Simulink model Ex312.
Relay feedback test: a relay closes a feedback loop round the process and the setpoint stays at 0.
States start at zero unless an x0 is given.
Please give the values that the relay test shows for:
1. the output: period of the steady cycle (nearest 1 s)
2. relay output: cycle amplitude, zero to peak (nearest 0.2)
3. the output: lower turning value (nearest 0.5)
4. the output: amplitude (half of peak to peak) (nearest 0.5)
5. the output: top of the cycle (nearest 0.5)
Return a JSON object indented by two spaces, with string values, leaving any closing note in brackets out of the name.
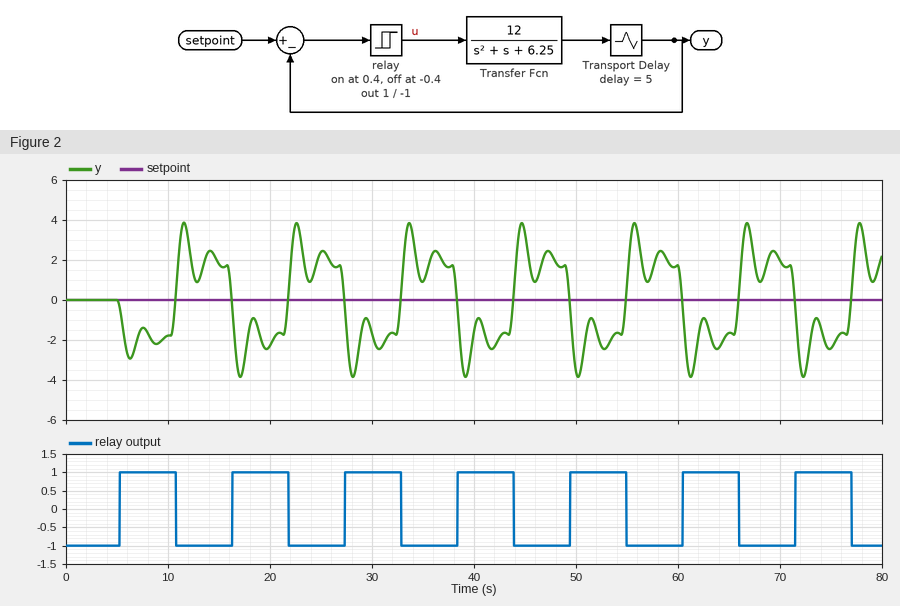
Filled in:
{
  "the output: period of the steady cycle": "11 s",
  "relay output: cycle amplitude, zero to peak": "1.0",
  "the output: lower turning value": "-4.0",
  "the output: amplitude (half of peak to peak)": "4.0",
  "the output: top of the cycle": "4.0"
}
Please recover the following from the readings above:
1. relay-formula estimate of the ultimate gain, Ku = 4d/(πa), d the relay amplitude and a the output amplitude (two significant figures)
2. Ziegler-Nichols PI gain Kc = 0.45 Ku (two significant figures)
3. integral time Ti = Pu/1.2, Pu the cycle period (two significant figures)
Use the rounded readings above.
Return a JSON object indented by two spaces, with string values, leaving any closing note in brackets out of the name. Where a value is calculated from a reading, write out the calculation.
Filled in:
{
  "relay-formula estimate of the ultimate gain, Ku = 4d/(πa), d the relay amplitude and a the output amplitude": "4 × 1 / (π × 4) = 0.32",
  "Ziegler-Nichols PI gain Kc = 0.45 Ku": "0.45 × 0.32 = 0.14",
  "integral time Ti = Pu/1.2, Pu the cycle period": "11 / 1.2 = 9.2 s"
}
